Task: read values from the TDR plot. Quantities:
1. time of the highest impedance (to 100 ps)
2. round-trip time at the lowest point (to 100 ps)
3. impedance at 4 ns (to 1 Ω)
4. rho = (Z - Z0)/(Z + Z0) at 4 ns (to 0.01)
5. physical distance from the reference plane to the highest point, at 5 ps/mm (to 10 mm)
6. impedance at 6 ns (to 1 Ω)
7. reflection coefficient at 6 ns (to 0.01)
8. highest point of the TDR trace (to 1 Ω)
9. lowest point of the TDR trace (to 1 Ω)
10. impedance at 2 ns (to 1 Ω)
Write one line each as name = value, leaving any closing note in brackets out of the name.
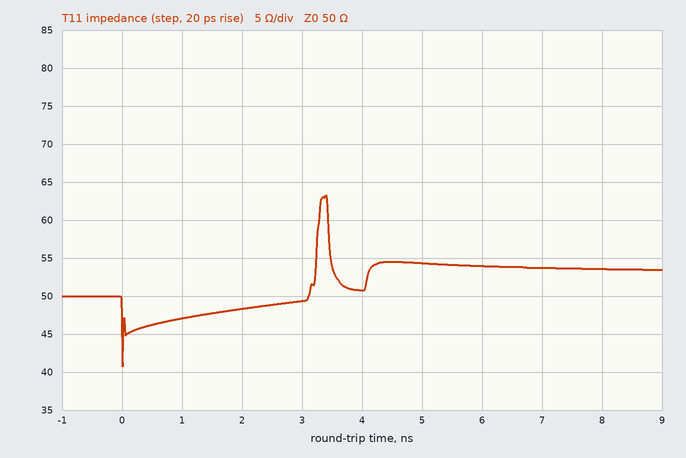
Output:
time of the highest impedance = 3.4 ns
round-trip time at the lowest point = 0.0 ns
impedance at 4 ns = 51 Ω
rho = (Z - Z0)/(Z + Z0) at 4 ns = +0.01
physical distance from the reference plane to the highest point, at 5 ps/mm = 340 mm
impedance at 6 ns = 54 Ω
reflection coefficient at 6 ns = +0.04
highest point of the TDR trace = 63 Ω
lowest point of the TDR trace = 41 Ω
impedance at 2 ns = 48 Ω
